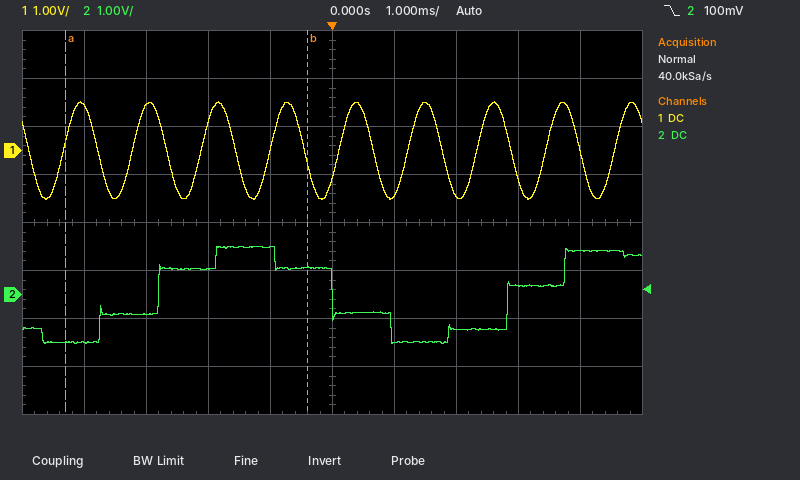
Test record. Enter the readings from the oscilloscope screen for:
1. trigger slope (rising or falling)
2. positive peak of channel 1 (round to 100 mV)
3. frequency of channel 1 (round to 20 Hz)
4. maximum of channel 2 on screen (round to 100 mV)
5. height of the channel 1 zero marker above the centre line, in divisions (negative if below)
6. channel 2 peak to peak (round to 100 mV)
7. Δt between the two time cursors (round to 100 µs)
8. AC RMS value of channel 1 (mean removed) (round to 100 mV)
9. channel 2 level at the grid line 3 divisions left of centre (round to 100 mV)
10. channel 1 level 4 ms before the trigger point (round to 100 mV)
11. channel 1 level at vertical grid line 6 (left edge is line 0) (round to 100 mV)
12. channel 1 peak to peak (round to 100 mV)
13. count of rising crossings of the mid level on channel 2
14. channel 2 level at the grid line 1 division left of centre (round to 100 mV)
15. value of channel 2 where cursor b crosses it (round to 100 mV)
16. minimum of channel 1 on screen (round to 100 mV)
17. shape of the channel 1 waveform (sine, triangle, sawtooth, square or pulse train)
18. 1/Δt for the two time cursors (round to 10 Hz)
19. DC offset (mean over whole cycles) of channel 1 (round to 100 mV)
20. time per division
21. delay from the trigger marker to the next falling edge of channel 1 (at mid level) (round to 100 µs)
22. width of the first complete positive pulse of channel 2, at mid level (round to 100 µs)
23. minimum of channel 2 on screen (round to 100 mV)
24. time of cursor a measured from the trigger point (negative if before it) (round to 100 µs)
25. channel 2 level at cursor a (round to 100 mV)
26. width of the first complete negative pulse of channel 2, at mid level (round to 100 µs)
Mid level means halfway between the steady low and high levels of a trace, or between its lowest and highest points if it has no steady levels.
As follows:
falling
1.0 V
900 Hz
1.0 V
+1.5 div
2.0 V
3.9 ms
700 mV
-400 mV
900 mV
-900 mV
2.0 V
2
1.0 V
600 mV
-1.0 V
sine
260 Hz
0.0 V
1 ms
700 µs
2.8 ms
-1.0 V
-4.3 ms
-1.0 V
2.8 ms
